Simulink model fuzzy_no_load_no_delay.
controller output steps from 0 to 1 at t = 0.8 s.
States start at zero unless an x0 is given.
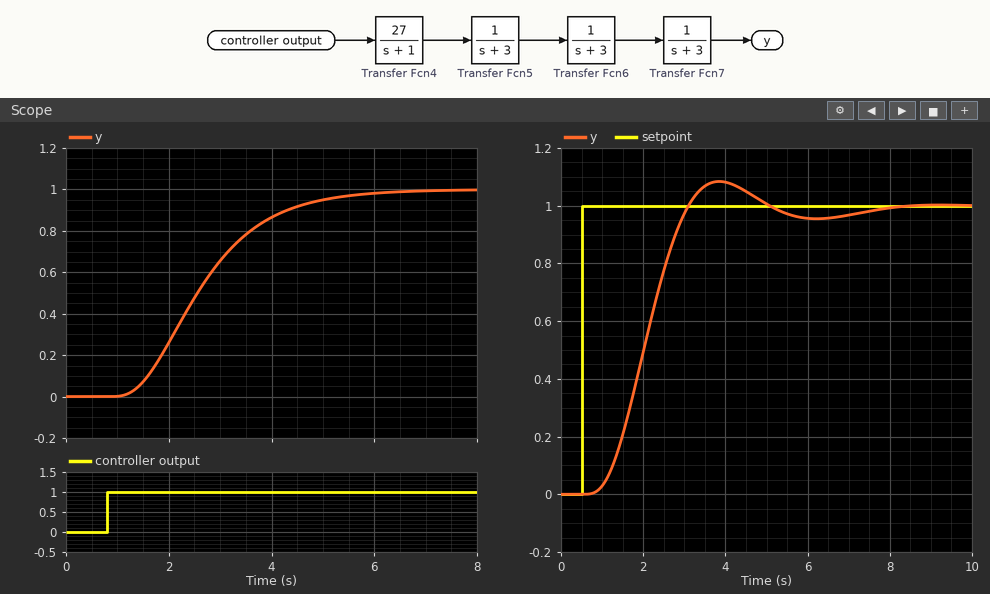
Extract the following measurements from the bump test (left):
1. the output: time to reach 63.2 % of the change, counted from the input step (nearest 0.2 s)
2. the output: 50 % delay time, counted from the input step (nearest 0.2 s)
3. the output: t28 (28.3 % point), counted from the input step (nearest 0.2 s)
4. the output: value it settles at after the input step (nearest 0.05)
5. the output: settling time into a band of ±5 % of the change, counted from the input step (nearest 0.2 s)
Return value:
2.2 s
1.8 s
1.2 s
1.00
4.2 s
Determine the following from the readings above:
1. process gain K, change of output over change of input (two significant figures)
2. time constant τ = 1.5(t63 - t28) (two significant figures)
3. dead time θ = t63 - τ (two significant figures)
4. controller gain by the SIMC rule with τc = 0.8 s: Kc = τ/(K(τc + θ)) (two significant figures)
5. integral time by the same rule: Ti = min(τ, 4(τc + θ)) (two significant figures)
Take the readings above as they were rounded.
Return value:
1.0
1.5 s
0.70 s
1.0
1.5 s
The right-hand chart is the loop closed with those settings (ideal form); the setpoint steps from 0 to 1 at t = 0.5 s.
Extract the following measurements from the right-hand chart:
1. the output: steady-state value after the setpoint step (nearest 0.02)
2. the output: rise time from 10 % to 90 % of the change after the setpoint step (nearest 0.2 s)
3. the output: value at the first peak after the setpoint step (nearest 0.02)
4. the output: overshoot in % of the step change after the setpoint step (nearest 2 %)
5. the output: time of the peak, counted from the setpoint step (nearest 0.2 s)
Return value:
1.00
1.6 s
1.08
8 %
3.4 s
